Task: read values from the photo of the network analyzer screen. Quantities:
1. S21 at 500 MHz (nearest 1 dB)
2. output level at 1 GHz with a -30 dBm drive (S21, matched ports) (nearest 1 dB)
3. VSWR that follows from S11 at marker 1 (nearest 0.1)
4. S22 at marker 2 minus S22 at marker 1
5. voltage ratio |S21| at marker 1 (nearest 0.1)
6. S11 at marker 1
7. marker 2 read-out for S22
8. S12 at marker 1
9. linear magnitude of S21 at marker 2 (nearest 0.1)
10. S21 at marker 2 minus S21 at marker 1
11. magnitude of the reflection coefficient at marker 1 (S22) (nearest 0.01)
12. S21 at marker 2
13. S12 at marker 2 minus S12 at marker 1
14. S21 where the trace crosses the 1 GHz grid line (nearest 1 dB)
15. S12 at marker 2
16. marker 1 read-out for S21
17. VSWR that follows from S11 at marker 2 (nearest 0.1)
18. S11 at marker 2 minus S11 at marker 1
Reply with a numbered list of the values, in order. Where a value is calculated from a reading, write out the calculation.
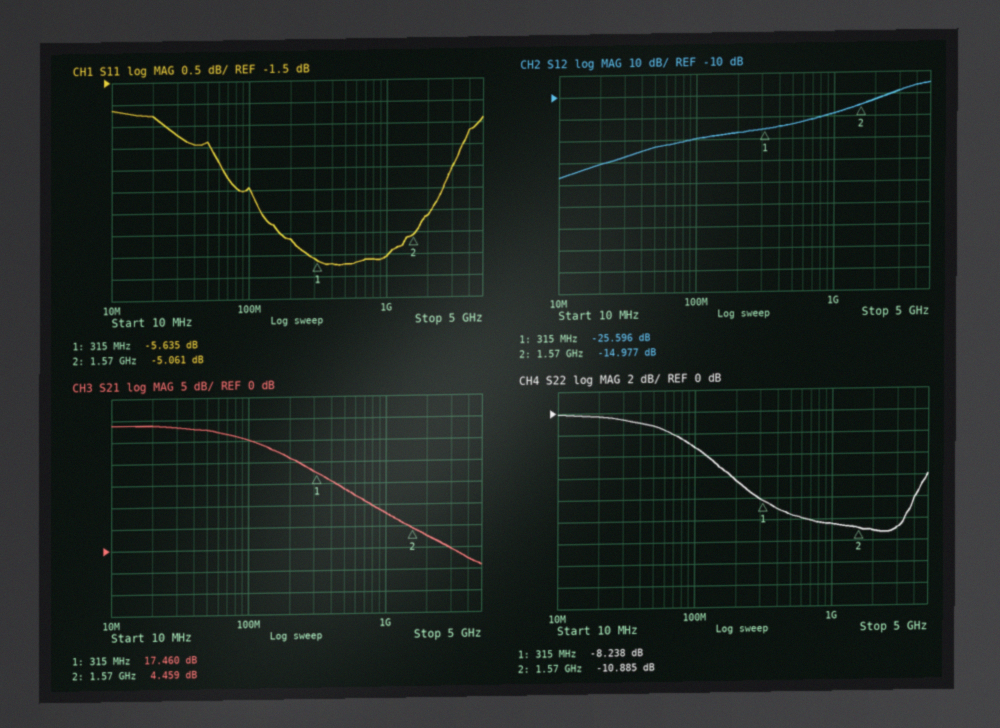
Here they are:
1. 14 dB
2. -30 dBm + (8 dB) = -22 dBm
3. (1 + 0.5227)/(1 − 0.5227) ≈ 3.2
4. -10.885 − (-8.238) = -2.647 dB
5. 10^(17.46/20) ≈ 7.5
6. -5.635 dB
7. -10.885 dB
8. -25.596 dB
9. 10^(4.459/20) ≈ 1.7
10. 4.459 − (17.46) = -13.001 dB
11. 10^(-8.238/20) ≈ 0.39
12. 4.459 dB
13. -14.977 − (-25.596) = 10.619 dB
14. 8 dB
15. -14.977 dB
16. 17.460 dB
17. (1 + 0.5584)/(1 − 0.5584) ≈ 3.5
18. -5.061 − (-5.635) = 0.574 dB
